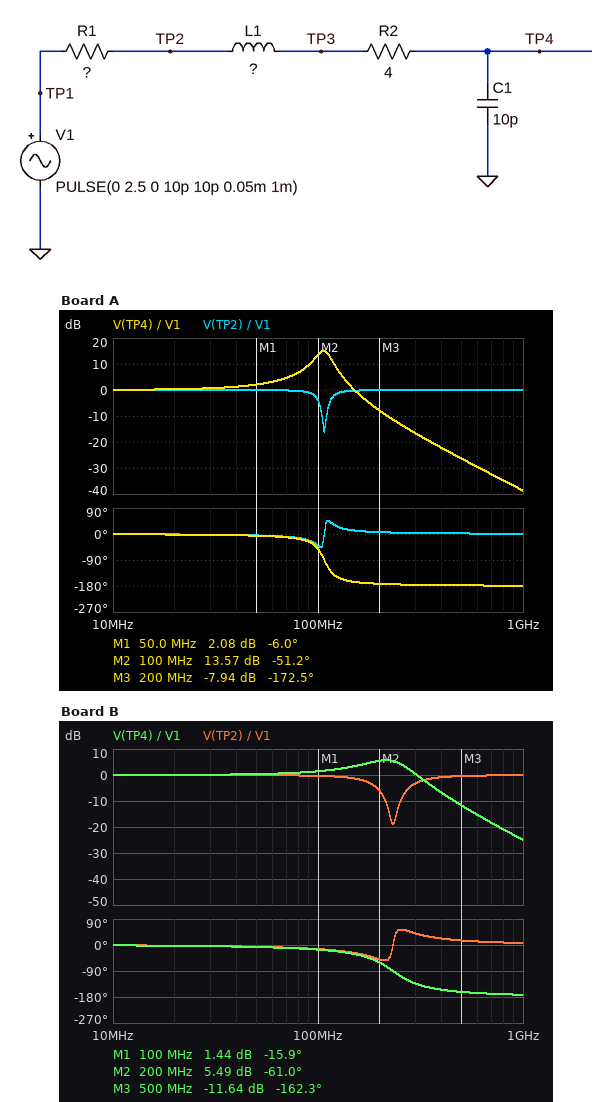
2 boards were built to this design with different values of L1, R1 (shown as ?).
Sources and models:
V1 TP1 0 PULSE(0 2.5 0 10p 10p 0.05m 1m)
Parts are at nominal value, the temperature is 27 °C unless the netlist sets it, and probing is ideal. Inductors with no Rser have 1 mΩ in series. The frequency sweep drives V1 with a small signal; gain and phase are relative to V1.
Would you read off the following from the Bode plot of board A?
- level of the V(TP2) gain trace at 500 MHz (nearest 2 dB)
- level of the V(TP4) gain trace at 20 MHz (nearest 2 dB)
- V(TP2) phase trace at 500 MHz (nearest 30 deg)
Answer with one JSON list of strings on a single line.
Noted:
["0 dB", "0 dB", "0 deg"]
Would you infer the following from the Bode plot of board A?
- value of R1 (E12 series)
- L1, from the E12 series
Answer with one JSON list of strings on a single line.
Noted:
["22 Ω", "220 nH"]
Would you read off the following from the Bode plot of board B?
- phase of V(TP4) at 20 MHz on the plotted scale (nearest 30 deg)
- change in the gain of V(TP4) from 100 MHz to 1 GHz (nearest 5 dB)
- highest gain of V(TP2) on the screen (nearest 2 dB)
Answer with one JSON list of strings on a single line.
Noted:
["0 deg", "-25 dB", "0 dB"]
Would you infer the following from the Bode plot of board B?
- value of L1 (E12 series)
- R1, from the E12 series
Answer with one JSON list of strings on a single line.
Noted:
["47 nH", "33 Ω"]
